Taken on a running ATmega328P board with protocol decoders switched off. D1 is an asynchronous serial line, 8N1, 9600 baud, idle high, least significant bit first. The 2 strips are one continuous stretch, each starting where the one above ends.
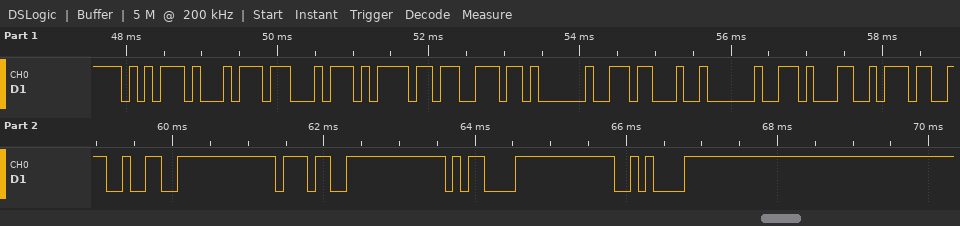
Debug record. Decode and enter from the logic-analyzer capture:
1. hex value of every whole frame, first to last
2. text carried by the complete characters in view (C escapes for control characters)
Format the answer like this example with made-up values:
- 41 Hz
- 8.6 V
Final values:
- 0x75 0x74 0x74 0x6F 0x6E 0x20 0x23 0x20 0x31 0x37 0x32 0x37 0x0D 0x0A
- "utton # 1727\r\n"
